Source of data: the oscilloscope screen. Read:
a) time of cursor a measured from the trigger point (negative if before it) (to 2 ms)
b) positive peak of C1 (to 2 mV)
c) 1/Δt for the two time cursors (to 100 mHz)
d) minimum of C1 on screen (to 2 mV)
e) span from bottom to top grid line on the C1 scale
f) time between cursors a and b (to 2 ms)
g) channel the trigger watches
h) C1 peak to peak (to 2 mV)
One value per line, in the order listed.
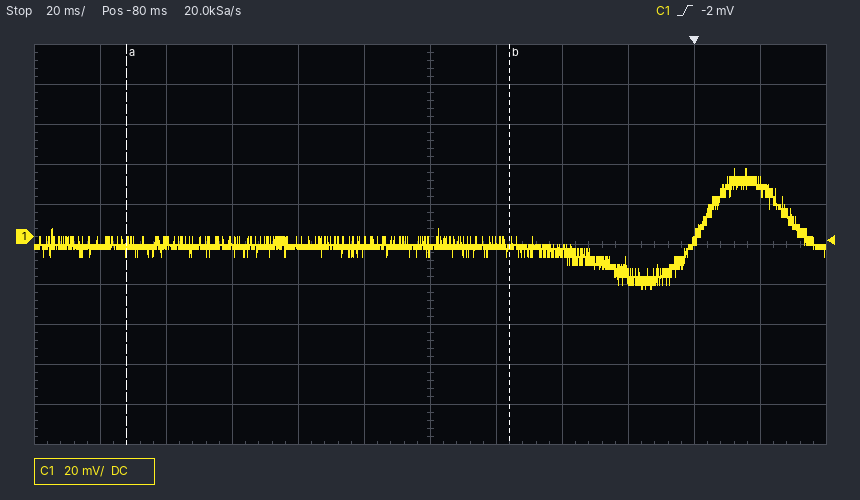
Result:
-172 ms
34 mV
8.6 Hz
-26 mV
200 mV
116 ms
C1
60 mV
